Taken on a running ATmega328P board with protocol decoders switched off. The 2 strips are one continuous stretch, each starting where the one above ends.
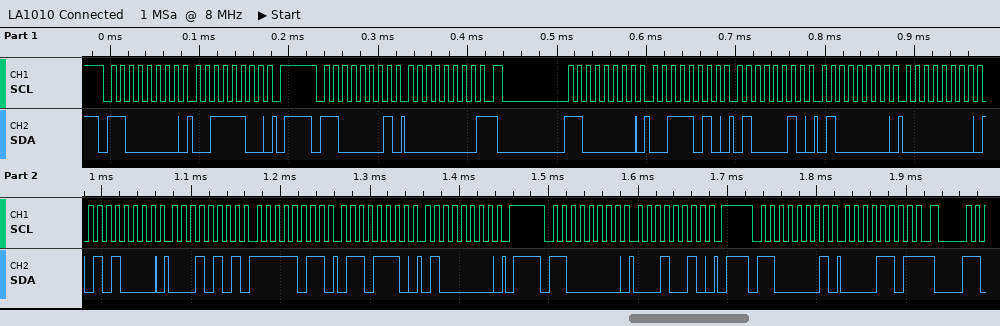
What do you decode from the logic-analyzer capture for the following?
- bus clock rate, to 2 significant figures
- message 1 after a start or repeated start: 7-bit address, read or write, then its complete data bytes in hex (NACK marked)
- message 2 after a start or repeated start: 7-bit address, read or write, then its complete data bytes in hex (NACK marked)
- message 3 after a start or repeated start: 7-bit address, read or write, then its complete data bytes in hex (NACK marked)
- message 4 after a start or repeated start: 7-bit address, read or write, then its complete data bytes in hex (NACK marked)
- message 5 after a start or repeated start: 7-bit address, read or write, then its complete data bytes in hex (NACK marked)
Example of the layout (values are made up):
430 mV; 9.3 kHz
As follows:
100 kHz; 0x60 write: 3C; 0x60 read: 00 NACK; 0x60 write: 3A 42 40 00 50 15 FB 6E 40; 0x60 write: 12; 0x60 read: 0D NACK
